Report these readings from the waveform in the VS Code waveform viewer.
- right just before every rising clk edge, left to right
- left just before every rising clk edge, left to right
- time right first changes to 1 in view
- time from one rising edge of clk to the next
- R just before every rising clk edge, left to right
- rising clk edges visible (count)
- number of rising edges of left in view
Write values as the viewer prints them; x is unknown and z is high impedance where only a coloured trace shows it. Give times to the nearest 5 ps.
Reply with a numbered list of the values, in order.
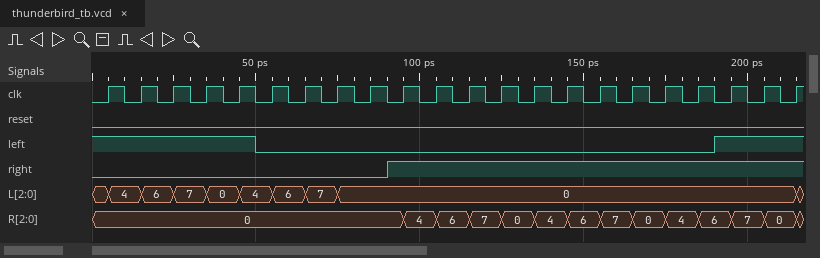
1. 0 0 0 0 0 0 0 0 0 1 1 1 1 1 1 1 1 1 1 1 1 1
2. 1 1 1 1 1 0 0 0 0 0 0 0 0 0 0 0 0 0 0 1 1 1
3. 90 ps
4. 10 ps
5. 0, 0, 0, 0, 0, 0, 0, 0, 0, 0, 4, 6, 7, 0, 4, 6, 7, 0, 4, 6, 7, 0
6. 22
7. 1
